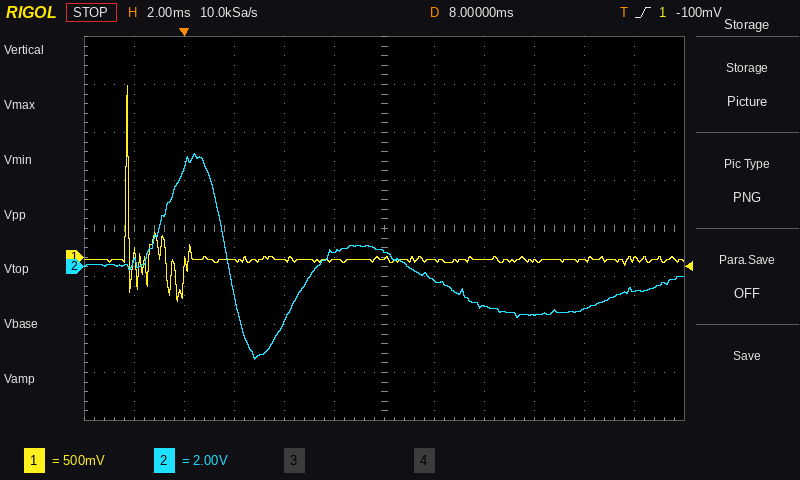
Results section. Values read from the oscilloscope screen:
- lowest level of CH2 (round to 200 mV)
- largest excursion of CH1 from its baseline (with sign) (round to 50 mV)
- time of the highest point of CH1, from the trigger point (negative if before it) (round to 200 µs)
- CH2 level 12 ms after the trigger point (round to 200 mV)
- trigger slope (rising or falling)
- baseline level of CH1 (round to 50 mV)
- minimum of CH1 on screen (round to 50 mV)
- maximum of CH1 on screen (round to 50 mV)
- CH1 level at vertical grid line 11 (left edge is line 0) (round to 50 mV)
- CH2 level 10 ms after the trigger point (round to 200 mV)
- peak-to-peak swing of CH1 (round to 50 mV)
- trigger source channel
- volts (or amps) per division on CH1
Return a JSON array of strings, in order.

["-3.8 V", "+1.80 V", "-2.2 ms", "-1.6 V", "rising", "0 mV", "-450 mV", "1.80 V", "0 mV", "-600 mV", "2.25 V", "CH1", "500 mV"]
